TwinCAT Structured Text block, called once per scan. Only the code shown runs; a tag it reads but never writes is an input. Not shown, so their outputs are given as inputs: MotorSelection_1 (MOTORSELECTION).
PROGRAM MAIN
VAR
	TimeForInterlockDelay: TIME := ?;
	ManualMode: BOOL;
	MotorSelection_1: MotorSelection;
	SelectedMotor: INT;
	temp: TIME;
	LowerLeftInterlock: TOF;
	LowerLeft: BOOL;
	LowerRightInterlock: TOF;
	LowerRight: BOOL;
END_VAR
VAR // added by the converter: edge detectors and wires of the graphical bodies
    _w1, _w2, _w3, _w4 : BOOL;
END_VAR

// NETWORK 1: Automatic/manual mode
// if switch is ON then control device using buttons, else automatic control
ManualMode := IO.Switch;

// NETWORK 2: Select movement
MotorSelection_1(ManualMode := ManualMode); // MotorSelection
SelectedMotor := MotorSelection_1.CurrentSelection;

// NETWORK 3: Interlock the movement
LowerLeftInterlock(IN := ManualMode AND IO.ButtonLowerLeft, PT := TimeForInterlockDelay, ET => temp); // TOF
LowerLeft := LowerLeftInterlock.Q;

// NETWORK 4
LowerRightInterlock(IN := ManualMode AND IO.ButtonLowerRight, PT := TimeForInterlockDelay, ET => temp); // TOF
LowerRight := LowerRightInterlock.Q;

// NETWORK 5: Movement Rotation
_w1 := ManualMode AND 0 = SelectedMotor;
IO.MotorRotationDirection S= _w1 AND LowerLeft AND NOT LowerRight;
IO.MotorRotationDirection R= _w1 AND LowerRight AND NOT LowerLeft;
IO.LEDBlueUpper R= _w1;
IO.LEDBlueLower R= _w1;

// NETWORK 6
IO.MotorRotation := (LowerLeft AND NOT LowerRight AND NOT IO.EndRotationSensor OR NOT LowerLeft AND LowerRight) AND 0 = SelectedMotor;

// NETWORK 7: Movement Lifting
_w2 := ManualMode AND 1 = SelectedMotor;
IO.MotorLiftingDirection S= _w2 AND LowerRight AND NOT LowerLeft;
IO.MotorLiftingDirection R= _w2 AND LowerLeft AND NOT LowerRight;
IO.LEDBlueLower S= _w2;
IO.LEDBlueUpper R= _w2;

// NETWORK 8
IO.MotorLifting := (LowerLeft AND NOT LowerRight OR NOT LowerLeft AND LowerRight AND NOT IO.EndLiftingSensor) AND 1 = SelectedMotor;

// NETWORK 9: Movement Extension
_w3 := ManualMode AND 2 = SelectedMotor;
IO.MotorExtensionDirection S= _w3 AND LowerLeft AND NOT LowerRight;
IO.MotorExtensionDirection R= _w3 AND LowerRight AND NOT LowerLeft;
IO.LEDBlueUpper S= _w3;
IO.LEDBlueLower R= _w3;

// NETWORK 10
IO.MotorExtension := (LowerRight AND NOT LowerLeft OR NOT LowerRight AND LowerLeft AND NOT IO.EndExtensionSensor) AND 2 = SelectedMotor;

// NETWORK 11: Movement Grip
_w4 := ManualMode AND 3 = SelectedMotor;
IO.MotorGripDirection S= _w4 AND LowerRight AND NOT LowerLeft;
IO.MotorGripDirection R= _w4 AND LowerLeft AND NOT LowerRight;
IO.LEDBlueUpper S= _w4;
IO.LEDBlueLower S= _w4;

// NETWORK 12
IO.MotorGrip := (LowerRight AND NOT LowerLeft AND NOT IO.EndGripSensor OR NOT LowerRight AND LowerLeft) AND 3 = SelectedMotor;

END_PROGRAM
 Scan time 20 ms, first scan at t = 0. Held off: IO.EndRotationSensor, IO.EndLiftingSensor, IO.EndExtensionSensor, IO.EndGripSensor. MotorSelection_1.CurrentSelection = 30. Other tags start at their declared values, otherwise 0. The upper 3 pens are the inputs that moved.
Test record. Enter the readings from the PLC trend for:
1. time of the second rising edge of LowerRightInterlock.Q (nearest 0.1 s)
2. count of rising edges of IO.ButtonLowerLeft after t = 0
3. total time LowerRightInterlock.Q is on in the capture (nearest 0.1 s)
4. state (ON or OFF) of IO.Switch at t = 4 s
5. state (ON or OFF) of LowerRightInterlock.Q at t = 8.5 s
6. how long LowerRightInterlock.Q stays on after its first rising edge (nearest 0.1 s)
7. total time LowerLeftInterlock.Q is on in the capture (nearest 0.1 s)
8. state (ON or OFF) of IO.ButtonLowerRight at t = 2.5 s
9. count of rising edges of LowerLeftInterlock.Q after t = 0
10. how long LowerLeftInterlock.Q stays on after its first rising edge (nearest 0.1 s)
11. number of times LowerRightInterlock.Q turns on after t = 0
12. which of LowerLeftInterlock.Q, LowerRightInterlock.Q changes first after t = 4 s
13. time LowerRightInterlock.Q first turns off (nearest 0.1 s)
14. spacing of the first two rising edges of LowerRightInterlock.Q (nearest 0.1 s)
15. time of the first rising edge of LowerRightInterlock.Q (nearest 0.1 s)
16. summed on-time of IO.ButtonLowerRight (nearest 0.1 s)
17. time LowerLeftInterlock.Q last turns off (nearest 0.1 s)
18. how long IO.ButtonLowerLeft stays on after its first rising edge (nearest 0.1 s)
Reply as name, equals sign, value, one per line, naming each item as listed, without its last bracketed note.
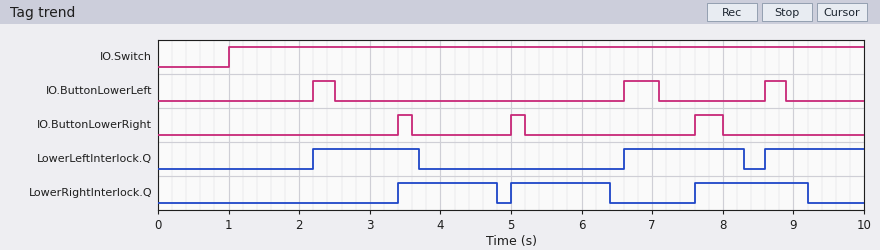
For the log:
time of the second rising edge of LowerRightInterlock.Q = 5.0 s
count of rising edges of IO.ButtonLowerLeft after t = 0 = 3
total time LowerRightInterlock.Q is on in the capture = 4.4 s
state (ON or OFF) of IO.Switch at t = 4 s = ON
state (ON or OFF) of LowerRightInterlock.Q at t = 8.5 s = ON
how long LowerRightInterlock.Q stays on after its first rising edge = 1.4 s
total time LowerLeftInterlock.Q is on in the capture = 4.6 s
state (ON or OFF) of IO.ButtonLowerRight at t = 2.5 s = OFF
count of rising edges of LowerLeftInterlock.Q after t = 0 = 3
how long LowerLeftInterlock.Q stays on after its first rising edge = 1.5 s
number of times LowerRightInterlock.Q turns on after t = 0 = 3
which of LowerLeftInterlock.Q, LowerRightInterlock.Q changes first after t = 4 s = LowerRightInterlock.Q
time LowerRightInterlock.Q first turns off = 4.8 s
spacing of the first two rising edges of LowerRightInterlock.Q = 1.6 s
time of the first rising edge of LowerRightInterlock.Q = 3.4 s
summed on-time of IO.ButtonLowerRight = 0.8 s
time LowerLeftInterlock.Q last turns off = 8.3 s
how long IO.ButtonLowerLeft stays on after its first rising edge = 0.3 s
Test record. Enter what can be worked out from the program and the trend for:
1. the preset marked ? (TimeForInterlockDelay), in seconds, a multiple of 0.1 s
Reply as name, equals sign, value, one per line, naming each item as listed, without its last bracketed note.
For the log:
the preset marked ? (TimeForInterlockDelay), in seconds, a multiple of 0.1 s = 1.2 s
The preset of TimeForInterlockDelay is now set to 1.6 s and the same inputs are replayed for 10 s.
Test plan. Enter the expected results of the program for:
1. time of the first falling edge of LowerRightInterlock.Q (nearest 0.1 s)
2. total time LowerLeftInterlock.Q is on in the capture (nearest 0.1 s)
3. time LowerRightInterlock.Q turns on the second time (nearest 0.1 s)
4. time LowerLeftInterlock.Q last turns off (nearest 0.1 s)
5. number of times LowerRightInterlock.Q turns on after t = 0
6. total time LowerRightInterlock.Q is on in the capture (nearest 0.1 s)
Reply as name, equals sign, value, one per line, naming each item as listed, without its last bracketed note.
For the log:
time of the first falling edge of LowerRightInterlock.Q = 6.8 s
total time LowerLeftInterlock.Q is on in the capture = 5.3 s
time LowerRightInterlock.Q turns on the second time = 7.6 s
time LowerLeftInterlock.Q last turns off = 4.1 s
number of times LowerRightInterlock.Q turns on after t = 0 = 2
total time LowerRightInterlock.Q is on in the capture = 5.4 s
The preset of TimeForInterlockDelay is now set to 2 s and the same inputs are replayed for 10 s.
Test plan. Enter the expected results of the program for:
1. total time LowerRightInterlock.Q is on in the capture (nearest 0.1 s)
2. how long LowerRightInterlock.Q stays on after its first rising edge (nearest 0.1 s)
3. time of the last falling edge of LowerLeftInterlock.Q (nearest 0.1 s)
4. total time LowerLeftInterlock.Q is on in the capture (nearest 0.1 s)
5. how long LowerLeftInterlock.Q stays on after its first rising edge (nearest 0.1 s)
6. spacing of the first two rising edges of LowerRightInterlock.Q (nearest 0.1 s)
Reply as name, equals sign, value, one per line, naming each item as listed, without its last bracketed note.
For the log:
total time LowerRightInterlock.Q is on in the capture = 6.2 s
how long LowerRightInterlock.Q stays on after its first rising edge = 3.8 s
time of the last falling edge of LowerLeftInterlock.Q = 4.5 s
total time LowerLeftInterlock.Q is on in the capture = 5.7 s
how long LowerLeftInterlock.Q stays on after its first rising edge = 2.3 s
spacing of the first two rising edges of LowerRightInterlock.Q = 4.2 s
